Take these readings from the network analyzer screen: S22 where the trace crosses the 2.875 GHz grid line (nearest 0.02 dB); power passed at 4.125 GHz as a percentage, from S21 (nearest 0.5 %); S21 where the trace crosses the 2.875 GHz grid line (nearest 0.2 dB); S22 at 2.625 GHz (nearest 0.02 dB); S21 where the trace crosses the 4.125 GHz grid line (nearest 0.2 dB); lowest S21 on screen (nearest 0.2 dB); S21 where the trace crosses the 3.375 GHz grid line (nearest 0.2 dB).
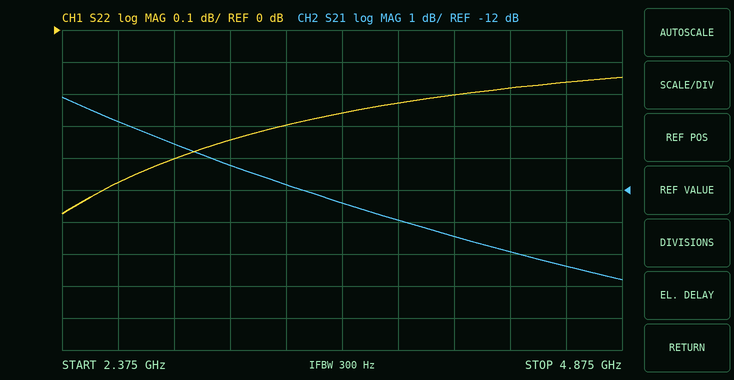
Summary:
-0.40 dB
4.5 %
-10.6 dB
-0.48 dB
-13.4 dB
-14.8 dB
-11.8 dB
